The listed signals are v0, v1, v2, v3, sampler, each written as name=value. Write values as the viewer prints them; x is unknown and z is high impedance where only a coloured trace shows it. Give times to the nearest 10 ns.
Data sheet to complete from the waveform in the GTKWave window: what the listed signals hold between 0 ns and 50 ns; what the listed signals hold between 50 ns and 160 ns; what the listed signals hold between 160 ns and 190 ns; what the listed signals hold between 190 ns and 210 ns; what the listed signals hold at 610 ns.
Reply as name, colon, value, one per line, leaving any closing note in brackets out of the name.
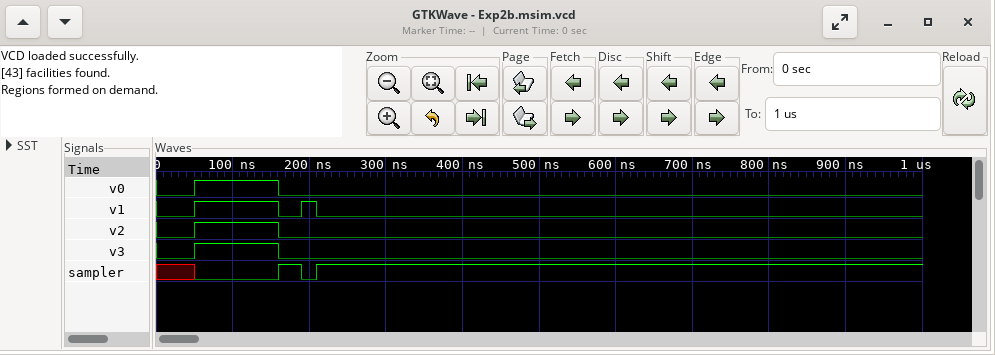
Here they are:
what the listed signals hold between 0 ns and 50 ns: v0=0, v1=0, v2=0, v3=0, sampler=x
what the listed signals hold between 50 ns and 160 ns: v0=1, v1=1, v2=1, v3=1, sampler=0
what the listed signals hold between 160 ns and 190 ns: v0=0, v1=0, v2=0, v3=0, sampler=1
what the listed signals hold between 190 ns and 210 ns: v0=0, v1=1, v2=0, v3=0, sampler=0
what the listed signals hold at 610 ns: v0=0, v1=0, v2=0, v3=0, sampler=1
